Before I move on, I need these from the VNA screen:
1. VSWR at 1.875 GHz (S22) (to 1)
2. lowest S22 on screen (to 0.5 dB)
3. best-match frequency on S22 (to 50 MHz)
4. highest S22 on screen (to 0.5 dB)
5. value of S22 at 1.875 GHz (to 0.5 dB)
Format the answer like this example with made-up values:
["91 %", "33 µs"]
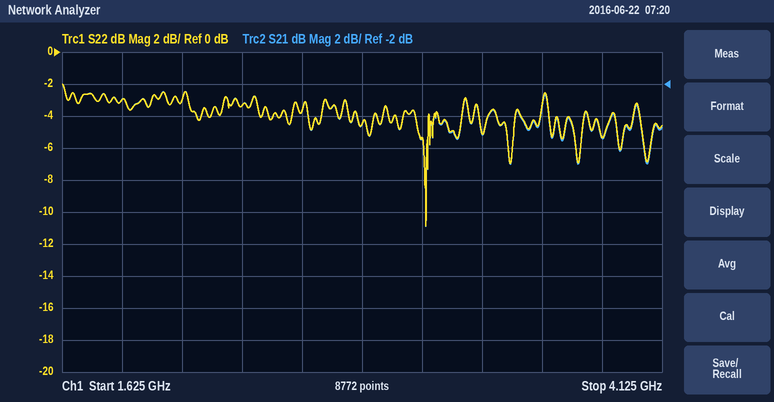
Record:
["6", "-11.0 dB", "3.15 GHz", "-2.0 dB", "-3.0 dB"]
